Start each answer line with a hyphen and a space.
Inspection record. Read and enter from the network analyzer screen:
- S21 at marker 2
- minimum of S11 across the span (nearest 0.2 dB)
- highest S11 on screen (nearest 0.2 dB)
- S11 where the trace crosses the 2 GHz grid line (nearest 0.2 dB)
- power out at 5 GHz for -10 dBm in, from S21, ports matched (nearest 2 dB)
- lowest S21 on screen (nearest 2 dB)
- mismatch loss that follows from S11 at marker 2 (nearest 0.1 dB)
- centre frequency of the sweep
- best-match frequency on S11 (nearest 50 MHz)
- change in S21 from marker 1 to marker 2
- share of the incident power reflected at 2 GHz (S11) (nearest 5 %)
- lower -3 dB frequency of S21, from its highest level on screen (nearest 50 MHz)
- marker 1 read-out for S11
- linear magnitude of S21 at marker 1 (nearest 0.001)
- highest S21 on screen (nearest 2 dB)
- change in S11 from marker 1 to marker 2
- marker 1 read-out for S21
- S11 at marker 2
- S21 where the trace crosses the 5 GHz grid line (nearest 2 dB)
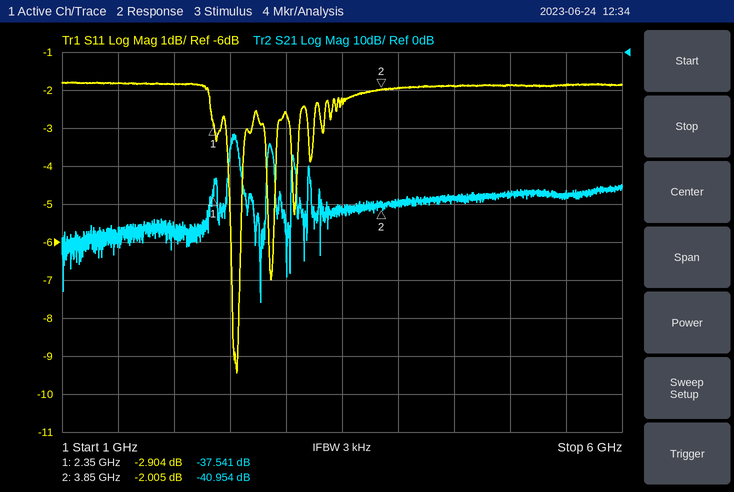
- -40.954 dB
- -9.4 dB
- -1.8 dB
- -1.8 dB
- -48 dBm
- -66 dB
- 4.3 dB
- 3.5 GHz
- 2.55 GHz
- -3.413 dB
- 65 %
- 2.50 GHz
- -2.904 dB
- 0.013
- -22 dB
- 0.899 dB
- -37.541 dB
- -2.005 dB
- -38 dB
